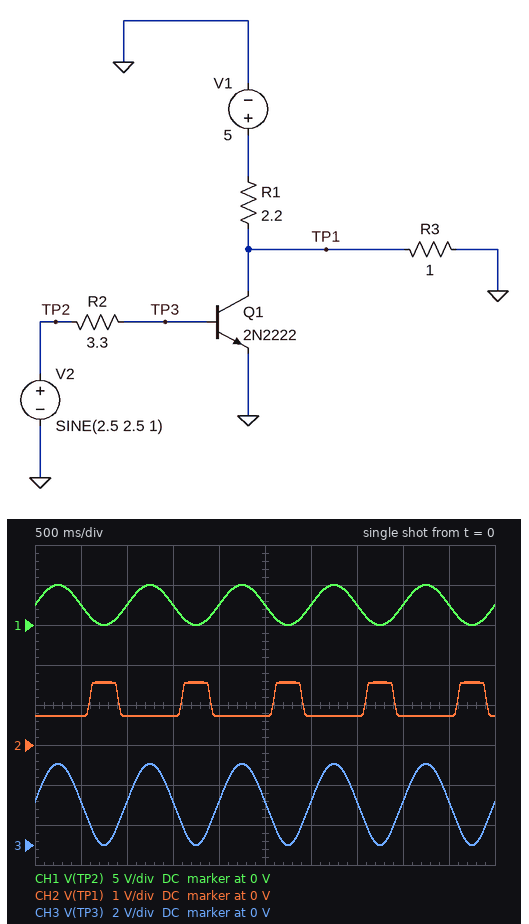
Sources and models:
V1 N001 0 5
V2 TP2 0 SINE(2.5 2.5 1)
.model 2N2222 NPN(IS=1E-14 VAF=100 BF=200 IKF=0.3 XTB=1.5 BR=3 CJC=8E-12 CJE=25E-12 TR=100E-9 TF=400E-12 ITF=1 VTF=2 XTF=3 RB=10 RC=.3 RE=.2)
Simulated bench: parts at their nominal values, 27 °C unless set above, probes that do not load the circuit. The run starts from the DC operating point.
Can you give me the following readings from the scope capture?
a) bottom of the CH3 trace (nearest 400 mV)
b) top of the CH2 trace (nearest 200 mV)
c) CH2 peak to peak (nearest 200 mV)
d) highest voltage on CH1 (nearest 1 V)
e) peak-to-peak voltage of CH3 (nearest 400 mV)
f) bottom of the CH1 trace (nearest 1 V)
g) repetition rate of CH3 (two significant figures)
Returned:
0 V
1.6 V
800 mV
5 V
4.0 V
0 V
1.0 Hz
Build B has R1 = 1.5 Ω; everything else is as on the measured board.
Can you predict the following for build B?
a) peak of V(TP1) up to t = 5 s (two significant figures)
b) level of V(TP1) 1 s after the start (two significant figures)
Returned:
2.0 V
990 mV
